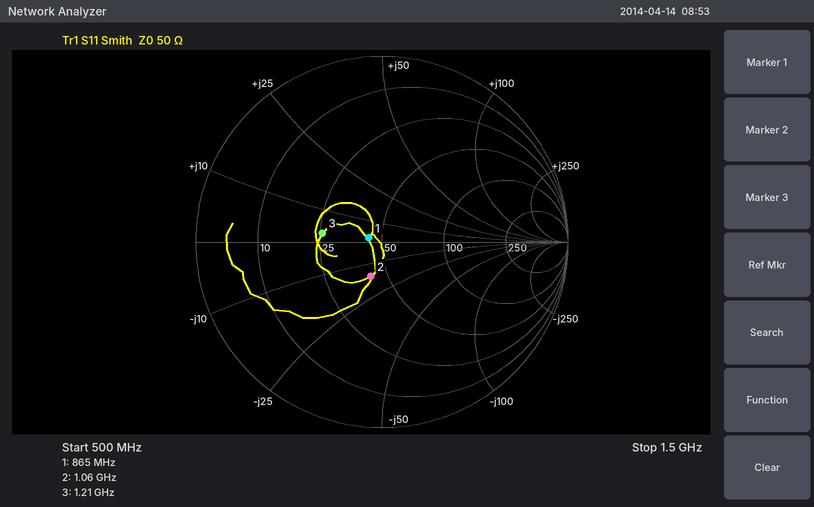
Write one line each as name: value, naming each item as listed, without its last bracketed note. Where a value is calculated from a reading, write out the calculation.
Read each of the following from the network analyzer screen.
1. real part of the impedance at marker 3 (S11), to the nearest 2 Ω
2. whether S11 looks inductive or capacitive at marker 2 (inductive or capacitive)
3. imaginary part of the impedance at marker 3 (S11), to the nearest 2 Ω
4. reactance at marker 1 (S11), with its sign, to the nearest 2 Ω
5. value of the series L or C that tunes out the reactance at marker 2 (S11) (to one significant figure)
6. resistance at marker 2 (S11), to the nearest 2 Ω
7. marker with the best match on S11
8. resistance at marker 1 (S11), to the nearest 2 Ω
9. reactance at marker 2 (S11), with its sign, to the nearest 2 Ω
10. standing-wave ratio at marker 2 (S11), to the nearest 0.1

real part of the impedance at marker 3 (S11), to the nearest 2 Ω: 26 Ω
whether S11 looks inductive or capacitive at marker 2: capacitive
imaginary part of the impedance at marker 3 (S11), to the nearest 2 Ω: +2 Ω
reactance at marker 1 (S11), with its sign, to the nearest 2 Ω: +2 Ω
value of the series L or C that tunes out the reactance at marker 2 (S11): L = 16 Ω/(2π × 1.06 GHz) ≈ 2 nH
resistance at marker 2 (S11), to the nearest 2 Ω: 42 Ω
marker with the best match on S11: marker 1
resistance at marker 1 (S11), to the nearest 2 Ω: 44 Ω
reactance at marker 2 (S11), with its sign, to the nearest 2 Ω: -16 Ω
standing-wave ratio at marker 2 (S11), to the nearest 0.1: 1.5
